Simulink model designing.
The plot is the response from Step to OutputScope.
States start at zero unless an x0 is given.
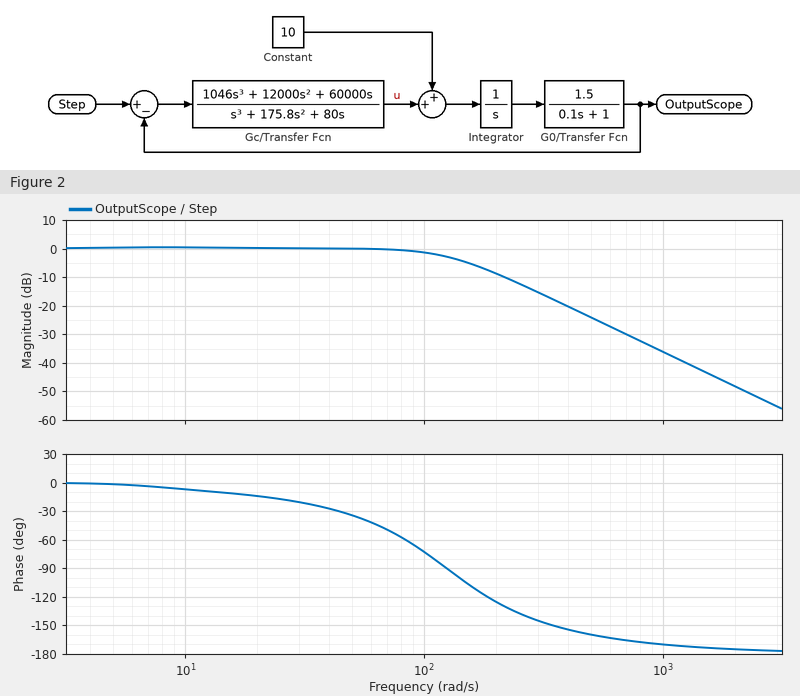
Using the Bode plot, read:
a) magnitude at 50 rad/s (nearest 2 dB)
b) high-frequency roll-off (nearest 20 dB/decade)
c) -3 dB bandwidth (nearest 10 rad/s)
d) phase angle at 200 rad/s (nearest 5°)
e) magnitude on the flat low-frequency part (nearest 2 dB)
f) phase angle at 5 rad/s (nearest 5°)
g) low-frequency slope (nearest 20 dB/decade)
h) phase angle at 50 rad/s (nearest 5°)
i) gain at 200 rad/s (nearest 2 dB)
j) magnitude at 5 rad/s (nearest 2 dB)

0 dB
-40 dB/decade
120 rad/s
-125°
0 dB
0°
0 dB/decade
-35°
-8 dB
0 dB
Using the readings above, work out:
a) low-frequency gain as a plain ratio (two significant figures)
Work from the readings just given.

1.0
